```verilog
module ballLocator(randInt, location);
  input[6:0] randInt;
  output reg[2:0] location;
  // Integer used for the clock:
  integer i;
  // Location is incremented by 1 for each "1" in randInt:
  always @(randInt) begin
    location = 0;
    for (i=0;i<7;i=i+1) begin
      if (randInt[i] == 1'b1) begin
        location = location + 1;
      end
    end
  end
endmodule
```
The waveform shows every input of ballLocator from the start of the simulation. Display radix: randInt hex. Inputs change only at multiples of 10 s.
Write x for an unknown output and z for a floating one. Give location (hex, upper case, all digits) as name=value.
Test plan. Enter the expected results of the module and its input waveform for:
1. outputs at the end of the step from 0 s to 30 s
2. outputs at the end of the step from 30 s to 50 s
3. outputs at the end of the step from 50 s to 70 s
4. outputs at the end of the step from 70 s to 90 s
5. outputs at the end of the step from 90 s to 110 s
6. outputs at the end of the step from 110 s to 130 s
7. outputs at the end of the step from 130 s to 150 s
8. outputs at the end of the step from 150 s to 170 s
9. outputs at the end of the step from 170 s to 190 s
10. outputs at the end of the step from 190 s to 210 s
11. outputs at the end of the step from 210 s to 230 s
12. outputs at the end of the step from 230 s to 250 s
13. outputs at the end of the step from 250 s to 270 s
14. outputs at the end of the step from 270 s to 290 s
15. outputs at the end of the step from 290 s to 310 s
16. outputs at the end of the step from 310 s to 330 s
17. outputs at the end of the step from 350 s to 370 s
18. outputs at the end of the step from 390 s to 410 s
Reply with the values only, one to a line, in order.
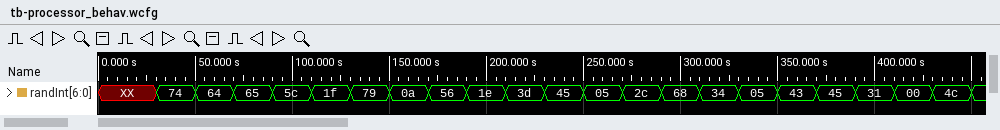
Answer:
location=x
location=4
location=3
location=4
location=4
location=5
location=5
location=2
location=4
location=4
location=5
location=3
location=2
location=3
location=3
location=3
location=3
location=3
